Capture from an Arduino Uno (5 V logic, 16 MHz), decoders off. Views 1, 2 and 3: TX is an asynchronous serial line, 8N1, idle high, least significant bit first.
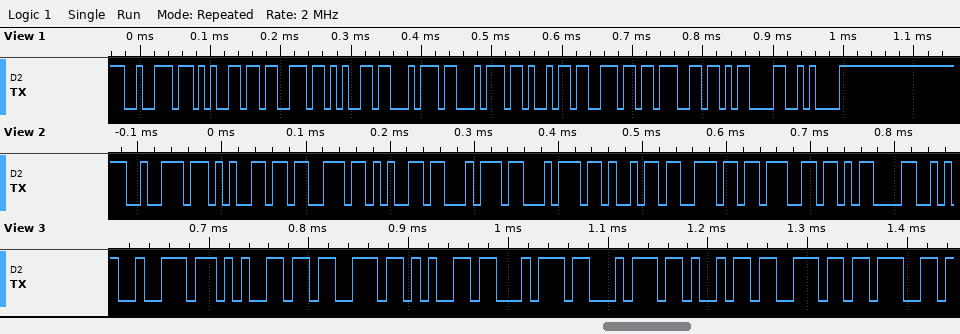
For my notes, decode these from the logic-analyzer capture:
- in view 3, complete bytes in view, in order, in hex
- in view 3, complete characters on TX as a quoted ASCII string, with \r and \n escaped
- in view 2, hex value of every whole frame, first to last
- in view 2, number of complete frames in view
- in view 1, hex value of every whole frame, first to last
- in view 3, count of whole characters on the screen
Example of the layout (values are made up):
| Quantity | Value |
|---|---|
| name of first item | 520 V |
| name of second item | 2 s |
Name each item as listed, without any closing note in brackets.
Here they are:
| Quantity | Value |
|---|---|
| in view 3, complete bytes in view, in order, in hex | 0x72 0x65 0x73 0x65 0x74 0x74 0x69 0x6E 0x67 |
| in view 3, complete characters on TX as a quoted ASCII string, with \r and \n escaped | "resetting" |
| in view 2, hex value of every whole frame, first to last | 72 65 73 65 74 74 69 6E 67 0D |
| in view 2, number of complete frames in view | 10 |
| in view 1, hex value of every whole frame, first to last | 72 65 73 65 74 74 69 6E 67 0D 0A |
| in view 3, count of whole characters on the screen | 9 |
